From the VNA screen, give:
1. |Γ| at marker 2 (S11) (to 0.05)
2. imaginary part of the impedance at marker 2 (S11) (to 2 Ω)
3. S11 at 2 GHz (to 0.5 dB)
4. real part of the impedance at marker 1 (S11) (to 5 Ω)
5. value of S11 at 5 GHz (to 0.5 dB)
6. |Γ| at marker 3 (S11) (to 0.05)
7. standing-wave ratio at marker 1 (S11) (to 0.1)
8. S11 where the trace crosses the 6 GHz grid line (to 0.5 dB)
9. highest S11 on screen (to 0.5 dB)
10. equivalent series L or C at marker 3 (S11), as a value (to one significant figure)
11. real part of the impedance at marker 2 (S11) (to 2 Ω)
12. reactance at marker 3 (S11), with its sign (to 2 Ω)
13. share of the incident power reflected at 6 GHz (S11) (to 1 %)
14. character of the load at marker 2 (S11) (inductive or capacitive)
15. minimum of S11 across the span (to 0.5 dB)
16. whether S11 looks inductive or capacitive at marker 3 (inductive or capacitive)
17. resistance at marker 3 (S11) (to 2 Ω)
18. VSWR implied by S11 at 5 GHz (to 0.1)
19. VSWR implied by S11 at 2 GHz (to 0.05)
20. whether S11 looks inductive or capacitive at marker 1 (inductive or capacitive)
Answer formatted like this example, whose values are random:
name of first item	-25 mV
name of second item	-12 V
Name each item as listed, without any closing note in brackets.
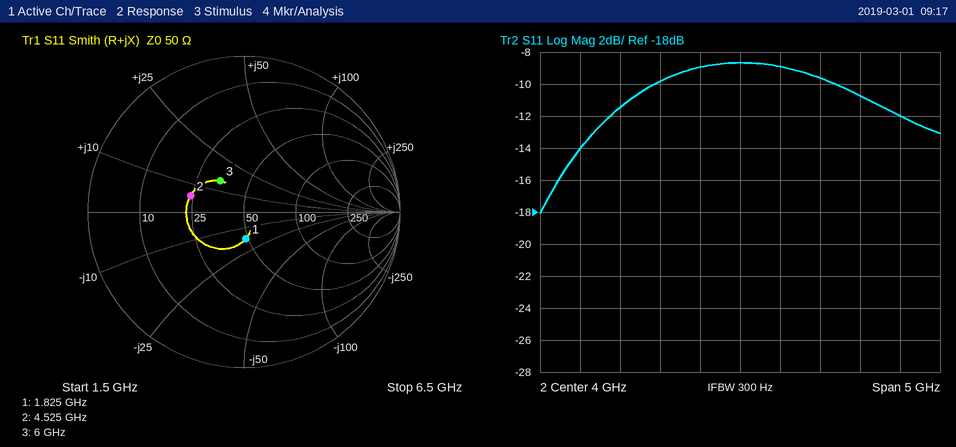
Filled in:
|Γ| at marker 2 (S11)	0.35
imaginary part of the impedance at marker 2 (S11)	+6 Ω
S11 at 2 GHz	-14.0 dB
real part of the impedance at marker 1 (S11)	50 Ω
value of S11 at 5 GHz	-9.5 dB
|Γ| at marker 3 (S11)	0.25
standing-wave ratio at marker 1 (S11)	1.4
S11 where the trace crosses the 6 GHz grid line	-12.0 dB
highest S11 on screen	-8.5 dB
equivalent series L or C at marker 3 (S11), as a value	400 pH
real part of the impedance at marker 2 (S11)	24 Ω
reactance at marker 3 (S11), with its sign	+14 Ω
share of the incident power reflected at 6 GHz (S11)	6 %
character of the load at marker 2 (S11)	inductive
minimum of S11 across the span	-18.0 dB
whether S11 looks inductive or capacitive at marker 3	inductive
resistance at marker 3 (S11)	34 Ω
VSWR implied by S11 at 5 GHz	2.0
VSWR implied by S11 at 2 GHz	1.50
whether S11 looks inductive or capacitive at marker 1	capacitive
